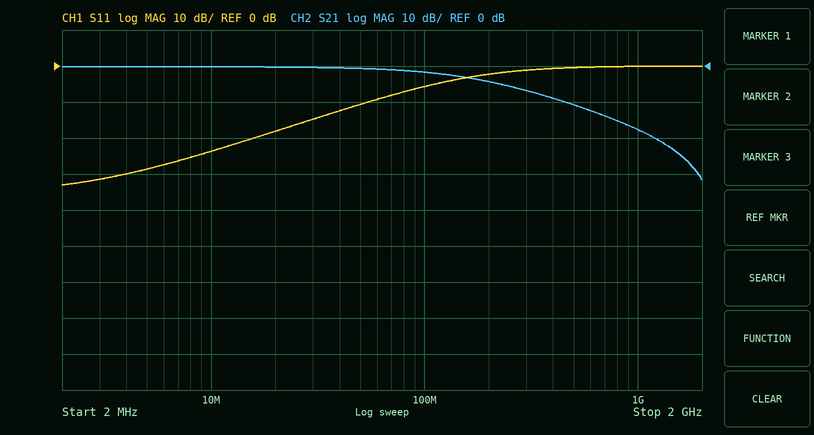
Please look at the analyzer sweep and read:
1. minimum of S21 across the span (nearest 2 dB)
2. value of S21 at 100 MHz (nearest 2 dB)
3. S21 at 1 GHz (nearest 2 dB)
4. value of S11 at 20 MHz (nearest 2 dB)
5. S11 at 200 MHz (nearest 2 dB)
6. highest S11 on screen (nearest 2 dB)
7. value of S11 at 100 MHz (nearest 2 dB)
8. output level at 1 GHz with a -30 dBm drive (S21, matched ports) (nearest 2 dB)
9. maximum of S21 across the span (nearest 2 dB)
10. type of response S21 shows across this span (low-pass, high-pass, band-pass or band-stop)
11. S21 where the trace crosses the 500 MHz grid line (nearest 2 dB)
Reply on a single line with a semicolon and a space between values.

-32 dB; -2 dB; -18 dB; -18 dB; -2 dB; 0 dB; -6 dB; -48 dBm; 0 dB; low-pass; -10 dB
